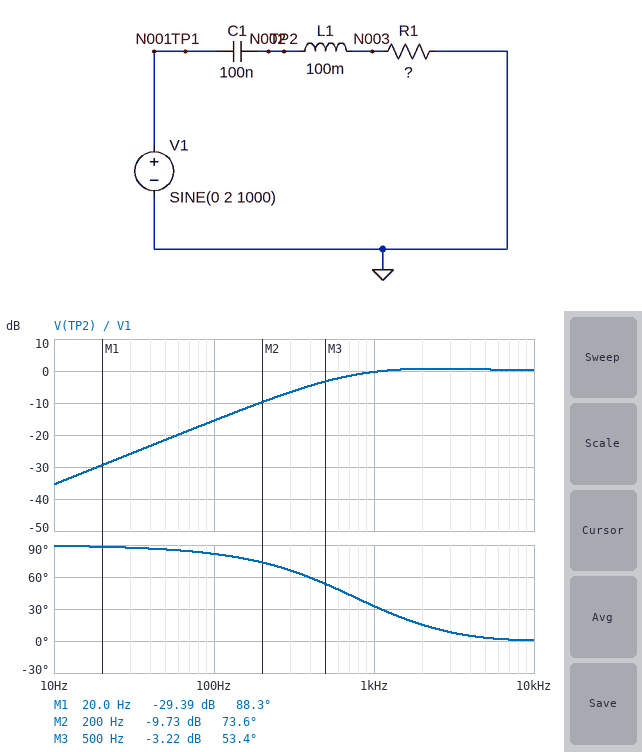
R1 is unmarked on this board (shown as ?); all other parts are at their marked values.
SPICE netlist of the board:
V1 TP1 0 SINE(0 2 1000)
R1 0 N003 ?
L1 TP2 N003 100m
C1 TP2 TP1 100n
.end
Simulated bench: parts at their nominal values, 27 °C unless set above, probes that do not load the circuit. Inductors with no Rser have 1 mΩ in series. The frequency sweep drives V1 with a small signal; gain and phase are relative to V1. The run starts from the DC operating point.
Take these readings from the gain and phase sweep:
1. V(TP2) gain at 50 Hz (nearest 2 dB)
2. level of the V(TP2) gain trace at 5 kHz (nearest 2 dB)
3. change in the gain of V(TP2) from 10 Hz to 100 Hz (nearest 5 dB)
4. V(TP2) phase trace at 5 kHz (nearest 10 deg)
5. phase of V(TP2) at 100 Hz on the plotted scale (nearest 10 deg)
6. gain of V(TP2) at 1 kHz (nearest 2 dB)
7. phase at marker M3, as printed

-22 dB
0 dB
20 dB
0 deg
80 deg
0 dB
53.4 deg
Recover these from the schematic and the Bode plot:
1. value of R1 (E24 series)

2.7 kΩ
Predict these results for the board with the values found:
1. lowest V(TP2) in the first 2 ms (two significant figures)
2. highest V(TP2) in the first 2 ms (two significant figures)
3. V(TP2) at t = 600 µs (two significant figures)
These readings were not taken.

-2.0 V
1.9 V
-1.9 V
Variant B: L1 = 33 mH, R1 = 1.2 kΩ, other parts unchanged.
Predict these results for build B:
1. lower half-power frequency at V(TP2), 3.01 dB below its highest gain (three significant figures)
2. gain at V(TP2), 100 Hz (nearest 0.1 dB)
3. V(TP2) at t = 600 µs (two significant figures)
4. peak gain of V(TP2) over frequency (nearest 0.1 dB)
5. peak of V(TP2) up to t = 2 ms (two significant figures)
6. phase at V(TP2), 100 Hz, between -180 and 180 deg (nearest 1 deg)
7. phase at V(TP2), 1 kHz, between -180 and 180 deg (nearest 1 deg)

1.32 kHz
-22.5 dB
-1.3 V
1.2 dB
1.3 V
87 deg
59 deg
